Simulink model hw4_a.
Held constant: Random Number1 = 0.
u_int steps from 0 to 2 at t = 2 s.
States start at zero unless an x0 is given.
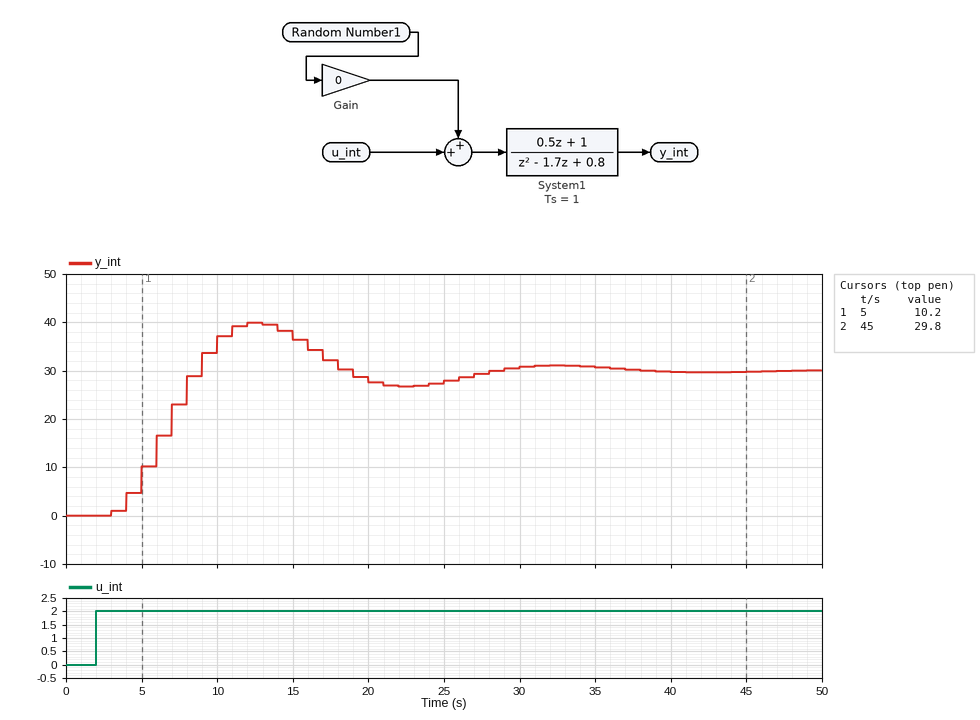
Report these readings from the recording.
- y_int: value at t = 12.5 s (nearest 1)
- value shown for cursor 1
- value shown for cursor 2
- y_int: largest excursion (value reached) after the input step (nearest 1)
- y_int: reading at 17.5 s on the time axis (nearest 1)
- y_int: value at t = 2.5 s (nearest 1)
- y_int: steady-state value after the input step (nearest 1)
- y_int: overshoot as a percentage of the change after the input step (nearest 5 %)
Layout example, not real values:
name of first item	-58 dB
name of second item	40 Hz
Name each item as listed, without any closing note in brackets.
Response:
y_int: value at t = 12.5 s	40
value shown for cursor 1	10.2
value shown for cursor 2	29.8
y_int: largest excursion (value reached) after the input step	40
y_int: reading at 17.5 s on the time axis	32
y_int: value at t = 2.5 s	0
y_int: steady-state value after the input step	30
y_int: overshoot as a percentage of the change after the input step	35 %
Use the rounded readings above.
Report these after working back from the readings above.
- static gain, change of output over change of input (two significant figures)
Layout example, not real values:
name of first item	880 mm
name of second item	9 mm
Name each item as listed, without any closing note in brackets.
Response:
static gain, change of output over change of input	15
